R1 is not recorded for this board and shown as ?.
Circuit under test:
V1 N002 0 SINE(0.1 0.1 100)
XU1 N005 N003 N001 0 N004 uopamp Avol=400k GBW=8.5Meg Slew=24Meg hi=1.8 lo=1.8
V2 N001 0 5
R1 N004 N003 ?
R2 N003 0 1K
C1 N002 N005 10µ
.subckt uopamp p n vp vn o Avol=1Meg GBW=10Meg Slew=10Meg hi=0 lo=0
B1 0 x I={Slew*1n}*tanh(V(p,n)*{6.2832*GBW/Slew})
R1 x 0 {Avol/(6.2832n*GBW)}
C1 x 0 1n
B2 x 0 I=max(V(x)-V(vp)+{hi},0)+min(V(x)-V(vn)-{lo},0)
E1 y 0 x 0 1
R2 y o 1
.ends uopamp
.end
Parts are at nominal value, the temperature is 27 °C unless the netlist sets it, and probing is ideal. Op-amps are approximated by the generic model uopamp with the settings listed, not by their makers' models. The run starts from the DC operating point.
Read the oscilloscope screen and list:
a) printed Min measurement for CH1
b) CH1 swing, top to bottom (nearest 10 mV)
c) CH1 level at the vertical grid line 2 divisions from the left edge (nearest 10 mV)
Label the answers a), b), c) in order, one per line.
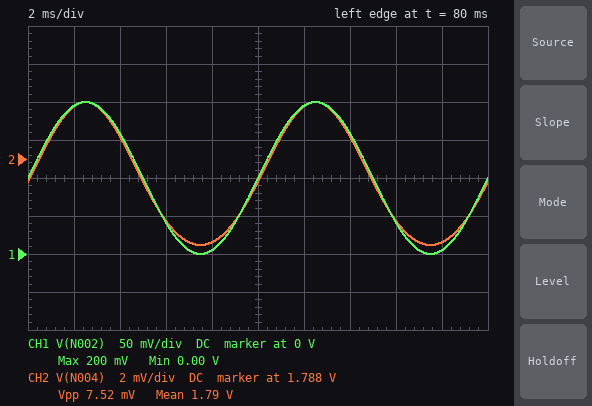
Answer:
a) 0.00 V
b) 200 mV
c) 160 mV
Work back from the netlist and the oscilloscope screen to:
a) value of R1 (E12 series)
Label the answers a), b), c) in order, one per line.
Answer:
a) 5.6 kΩ
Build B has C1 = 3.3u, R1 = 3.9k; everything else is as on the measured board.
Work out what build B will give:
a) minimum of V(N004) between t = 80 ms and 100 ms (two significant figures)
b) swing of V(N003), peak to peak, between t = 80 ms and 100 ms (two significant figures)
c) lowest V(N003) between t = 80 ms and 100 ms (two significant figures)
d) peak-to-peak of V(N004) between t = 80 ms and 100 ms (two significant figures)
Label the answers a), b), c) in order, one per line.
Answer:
a) 1.8 V
b) 1.2 mV
c) 360 mV
d) 5.9 mV
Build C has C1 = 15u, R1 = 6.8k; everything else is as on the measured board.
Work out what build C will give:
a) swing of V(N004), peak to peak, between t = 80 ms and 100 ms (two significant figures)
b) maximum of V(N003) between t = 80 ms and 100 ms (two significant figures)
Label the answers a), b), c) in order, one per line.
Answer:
a) 8.2 mV
b) 230 mV
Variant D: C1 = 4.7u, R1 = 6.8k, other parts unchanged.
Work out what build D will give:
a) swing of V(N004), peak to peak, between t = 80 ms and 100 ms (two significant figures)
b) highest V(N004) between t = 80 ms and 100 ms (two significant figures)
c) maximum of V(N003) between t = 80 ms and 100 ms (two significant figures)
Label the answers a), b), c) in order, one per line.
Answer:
a) 8.2 mV
b) 1.8 V
c) 230 mV
